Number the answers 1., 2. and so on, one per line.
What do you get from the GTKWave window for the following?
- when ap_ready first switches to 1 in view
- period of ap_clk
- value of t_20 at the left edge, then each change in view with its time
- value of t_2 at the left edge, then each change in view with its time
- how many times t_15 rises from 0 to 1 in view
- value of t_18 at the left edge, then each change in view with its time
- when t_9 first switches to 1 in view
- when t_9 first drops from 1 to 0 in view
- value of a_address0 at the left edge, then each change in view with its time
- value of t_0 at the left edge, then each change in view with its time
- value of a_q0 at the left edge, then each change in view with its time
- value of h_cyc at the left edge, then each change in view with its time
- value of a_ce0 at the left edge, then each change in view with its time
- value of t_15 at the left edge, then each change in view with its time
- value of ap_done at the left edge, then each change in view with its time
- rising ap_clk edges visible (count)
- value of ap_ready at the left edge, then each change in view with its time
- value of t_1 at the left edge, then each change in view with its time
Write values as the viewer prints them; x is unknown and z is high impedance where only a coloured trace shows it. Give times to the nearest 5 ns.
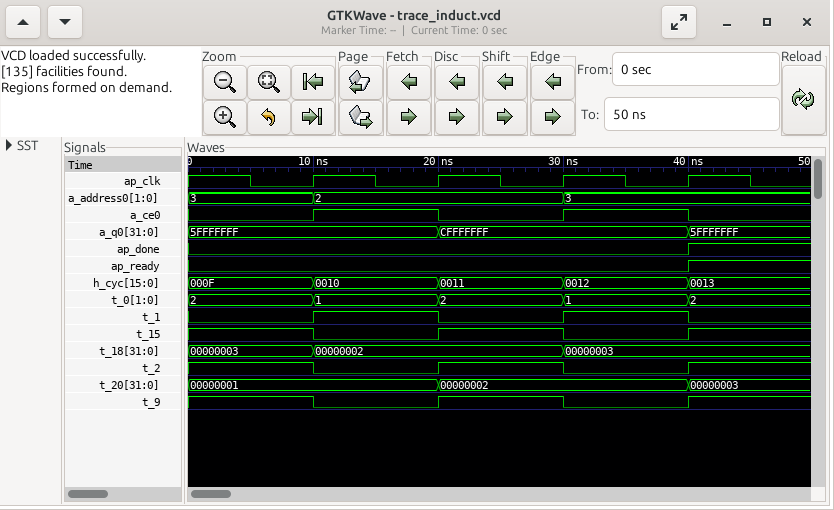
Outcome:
1. 40 ns
2. 10 ns
3. 00000001, 00000002 at 20 ns, 00000003 at 40 ns
4. 1, 0 at 10 ns, 1 at 20 ns, 0 at 30 ns, 1 at 40 ns
5. 2
6. 00000003, 00000002 at 10 ns, 00000003 at 30 ns
7. 20 ns
8. 10 ns
9. 3, 2 at 10 ns, 3 at 30 ns
10. 2, 1 at 10 ns, 2 at 20 ns, 1 at 30 ns, 2 at 40 ns
11. 5FFFFFFF, CFFFFFFF at 20 ns, 5FFFFFFF at 40 ns
12. 000F, 0010 at 10 ns, 0011 at 20 ns, 0012 at 30 ns, 0013 at 40 ns
13. 0, 1 at 10 ns, 0 at 20 ns, 1 at 30 ns, 0 at 40 ns
14. 1, 0 at 10 ns, 1 at 20 ns, 0 at 30 ns, 1 at 40 ns
15. 0, 1 at 40 ns
16. 4
17. 0, 1 at 40 ns
18. 0, 1 at 10 ns, 0 at 20 ns, 1 at 30 ns, 0 at 40 ns
